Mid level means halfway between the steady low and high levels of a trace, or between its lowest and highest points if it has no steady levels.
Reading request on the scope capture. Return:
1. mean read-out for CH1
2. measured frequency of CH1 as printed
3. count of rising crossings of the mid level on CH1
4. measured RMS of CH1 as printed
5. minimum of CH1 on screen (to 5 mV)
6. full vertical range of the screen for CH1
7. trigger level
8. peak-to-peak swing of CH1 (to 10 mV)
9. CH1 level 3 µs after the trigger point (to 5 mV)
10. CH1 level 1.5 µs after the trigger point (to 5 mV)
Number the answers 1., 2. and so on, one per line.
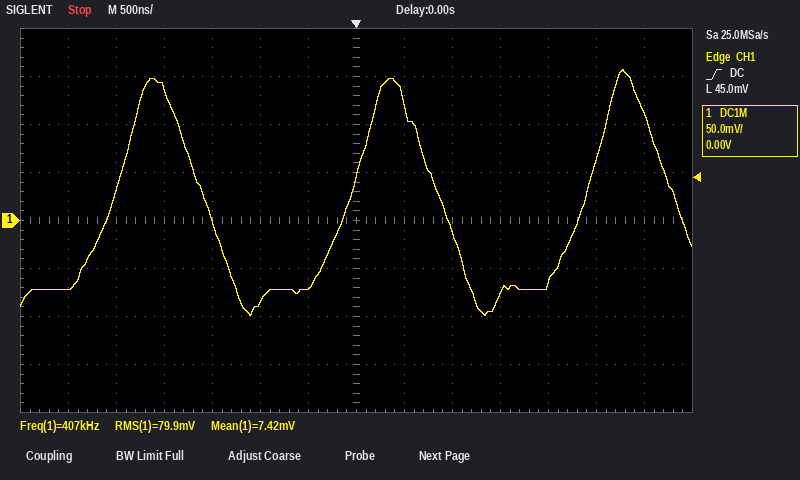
1. 7.42 mV
2. 407 kHz
3. 3
4. 79.9 mV
5. -100 mV
6. 400 mV
7. 45.0 mV
8. 260 mV
9. 110 mV
10. -75 mV
